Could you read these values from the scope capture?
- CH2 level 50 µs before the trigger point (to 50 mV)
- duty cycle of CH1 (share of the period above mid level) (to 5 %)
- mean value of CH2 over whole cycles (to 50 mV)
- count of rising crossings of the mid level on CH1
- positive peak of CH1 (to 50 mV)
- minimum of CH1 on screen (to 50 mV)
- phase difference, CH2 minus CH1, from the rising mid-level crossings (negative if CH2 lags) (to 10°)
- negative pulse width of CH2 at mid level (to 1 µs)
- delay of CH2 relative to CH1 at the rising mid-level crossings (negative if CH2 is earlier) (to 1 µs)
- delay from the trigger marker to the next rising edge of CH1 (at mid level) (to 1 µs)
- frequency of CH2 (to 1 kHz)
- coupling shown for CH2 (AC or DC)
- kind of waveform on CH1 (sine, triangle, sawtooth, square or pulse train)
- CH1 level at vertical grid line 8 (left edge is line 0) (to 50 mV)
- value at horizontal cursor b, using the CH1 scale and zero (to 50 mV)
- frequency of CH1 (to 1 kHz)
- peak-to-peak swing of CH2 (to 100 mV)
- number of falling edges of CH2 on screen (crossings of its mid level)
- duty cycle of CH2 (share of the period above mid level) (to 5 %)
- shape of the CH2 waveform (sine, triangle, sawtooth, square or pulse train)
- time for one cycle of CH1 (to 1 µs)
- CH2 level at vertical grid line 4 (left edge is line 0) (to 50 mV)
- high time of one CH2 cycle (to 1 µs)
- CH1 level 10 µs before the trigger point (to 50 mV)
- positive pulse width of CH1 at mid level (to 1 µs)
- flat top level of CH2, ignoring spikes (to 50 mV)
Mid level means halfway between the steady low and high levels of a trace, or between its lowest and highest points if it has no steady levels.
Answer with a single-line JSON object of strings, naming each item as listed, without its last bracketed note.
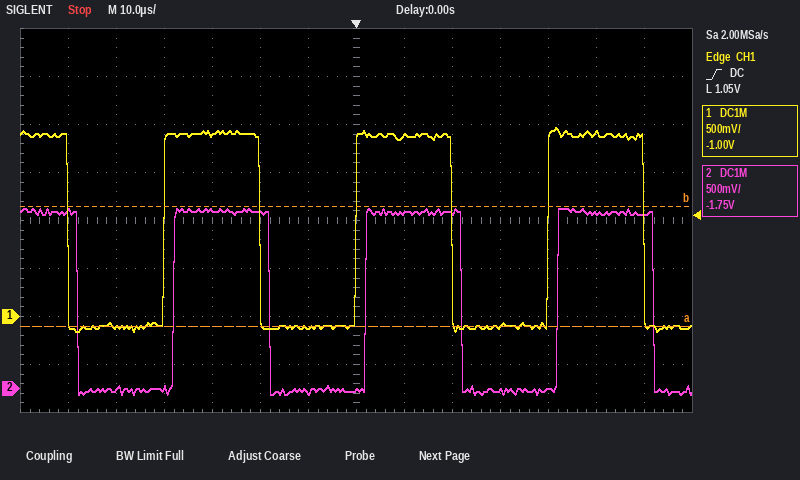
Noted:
{"CH2 level 50 µs before the trigger point": "0 mV", "duty cycle of CH1 (share of the period above mid level)": "50 %", "mean value of CH2 over whole cycles": "900 mV", "count of rising crossings of the mid level on CH1": "3", "positive peak of CH1": "1.95 V", "minimum of CH1 on screen": "-150 mV", "phase difference, CH2 minus CH1, from the rising mid-level crossings (negative if CH2 lags)": "-20°", "negative pulse width of CH2 at mid level": "20 µs", "delay of CH2 relative to CH1 at the rising mid-level crossings (negative if CH2 is earlier)": "+2 µs", "delay from the trigger marker to the next rising edge of CH1 (at mid level)": "40 µs", "frequency of CH2": "25 kHz", "coupling shown for CH2": "DC", "kind of waveform on CH1": "square", "CH1 level at vertical grid line 8 (left edge is line 0)": "1.90 V", "value at horizontal cursor b, using the CH1 scale and zero": "1.15 V", "frequency of CH1": "25 kHz", "peak-to-peak swing of CH2": "1.90 V", "number of falling edges of CH2 on screen": "4", "duty cycle of CH2 (share of the period above mid level)": "50 %", "shape of the CH2 waveform": "square", "time for one cycle of CH1": "40 µs", "CH2 level at vertical grid line 4 (left edge is line 0)": "1.85 V", "high time of one CH2 cycle": "20 µs", "CH1 level 10 µs before the trigger point": "-100 mV", "positive pulse width of CH1 at mid level": "20 µs", "flat top level of CH2, ignoring spikes": "1.85 V"}
